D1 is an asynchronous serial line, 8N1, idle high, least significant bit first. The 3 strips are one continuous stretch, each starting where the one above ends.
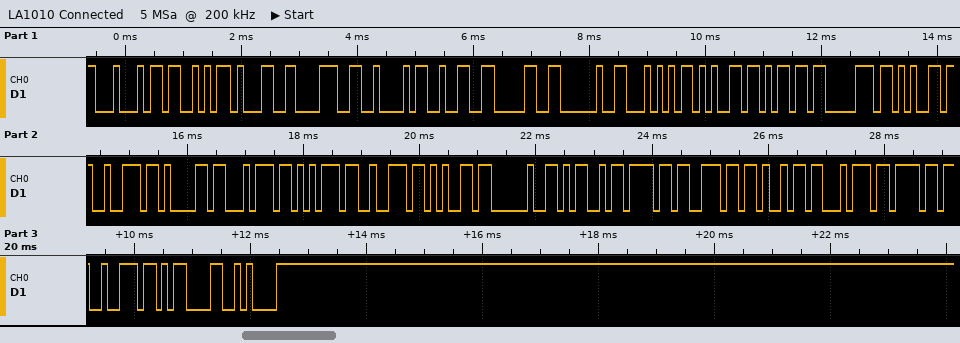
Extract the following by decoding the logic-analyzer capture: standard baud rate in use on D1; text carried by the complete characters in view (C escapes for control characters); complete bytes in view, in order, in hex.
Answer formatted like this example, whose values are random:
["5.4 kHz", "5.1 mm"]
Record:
["9600 baud", "\"DS18B20 Temperature Monitor\\r\\n\"", "44 53 31 38 42 32 30 20 54 65 6D 70 65 72 61 74 75 72 65 20 4D 6F 6E 69 74 6F 72 0D 0A"]
